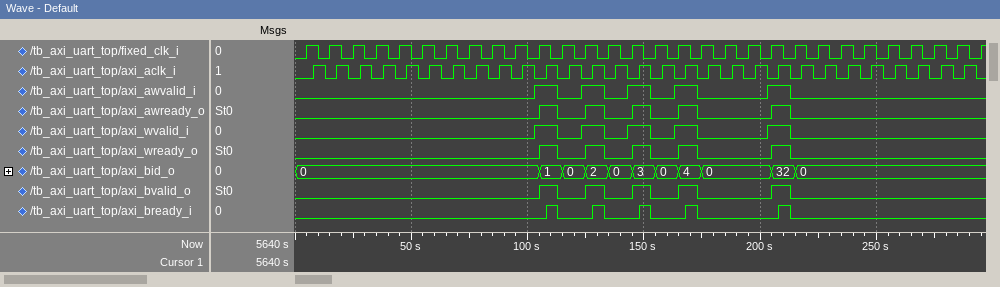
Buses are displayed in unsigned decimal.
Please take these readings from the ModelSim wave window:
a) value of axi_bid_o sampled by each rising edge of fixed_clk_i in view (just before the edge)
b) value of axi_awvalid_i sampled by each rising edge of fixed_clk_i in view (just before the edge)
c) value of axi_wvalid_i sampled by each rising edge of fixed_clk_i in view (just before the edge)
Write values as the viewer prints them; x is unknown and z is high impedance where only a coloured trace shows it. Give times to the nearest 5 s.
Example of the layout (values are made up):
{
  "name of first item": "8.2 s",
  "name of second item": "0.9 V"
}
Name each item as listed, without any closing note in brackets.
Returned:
{
  "value of axi_bid_o sampled by each rising edge of fixed_clk_i in view": "0, 0, 0, 0, 0, 0, 0, 0, 0, 0, 0, 1, 0, 2, 0, 3, 0, 4, 0, 0, 0, 32, 0, 0, 0, 0, 0, 0, 0, 0",
  "value of axi_awvalid_i sampled by each rising edge of fixed_clk_i in view": "0 0 0 0 0 0 0 0 0 0 1 0 1 0 1 0 1 0 0 0 1 0 0 0 0 0 0 0 0 0",
  "value of axi_wvalid_i sampled by each rising edge of fixed_clk_i in view": "0 0 0 0 0 0 0 0 0 0 1 0 1 0 1 0 1 0 0 0 1 0 0 0 0 0 0 0 0 0"
}
